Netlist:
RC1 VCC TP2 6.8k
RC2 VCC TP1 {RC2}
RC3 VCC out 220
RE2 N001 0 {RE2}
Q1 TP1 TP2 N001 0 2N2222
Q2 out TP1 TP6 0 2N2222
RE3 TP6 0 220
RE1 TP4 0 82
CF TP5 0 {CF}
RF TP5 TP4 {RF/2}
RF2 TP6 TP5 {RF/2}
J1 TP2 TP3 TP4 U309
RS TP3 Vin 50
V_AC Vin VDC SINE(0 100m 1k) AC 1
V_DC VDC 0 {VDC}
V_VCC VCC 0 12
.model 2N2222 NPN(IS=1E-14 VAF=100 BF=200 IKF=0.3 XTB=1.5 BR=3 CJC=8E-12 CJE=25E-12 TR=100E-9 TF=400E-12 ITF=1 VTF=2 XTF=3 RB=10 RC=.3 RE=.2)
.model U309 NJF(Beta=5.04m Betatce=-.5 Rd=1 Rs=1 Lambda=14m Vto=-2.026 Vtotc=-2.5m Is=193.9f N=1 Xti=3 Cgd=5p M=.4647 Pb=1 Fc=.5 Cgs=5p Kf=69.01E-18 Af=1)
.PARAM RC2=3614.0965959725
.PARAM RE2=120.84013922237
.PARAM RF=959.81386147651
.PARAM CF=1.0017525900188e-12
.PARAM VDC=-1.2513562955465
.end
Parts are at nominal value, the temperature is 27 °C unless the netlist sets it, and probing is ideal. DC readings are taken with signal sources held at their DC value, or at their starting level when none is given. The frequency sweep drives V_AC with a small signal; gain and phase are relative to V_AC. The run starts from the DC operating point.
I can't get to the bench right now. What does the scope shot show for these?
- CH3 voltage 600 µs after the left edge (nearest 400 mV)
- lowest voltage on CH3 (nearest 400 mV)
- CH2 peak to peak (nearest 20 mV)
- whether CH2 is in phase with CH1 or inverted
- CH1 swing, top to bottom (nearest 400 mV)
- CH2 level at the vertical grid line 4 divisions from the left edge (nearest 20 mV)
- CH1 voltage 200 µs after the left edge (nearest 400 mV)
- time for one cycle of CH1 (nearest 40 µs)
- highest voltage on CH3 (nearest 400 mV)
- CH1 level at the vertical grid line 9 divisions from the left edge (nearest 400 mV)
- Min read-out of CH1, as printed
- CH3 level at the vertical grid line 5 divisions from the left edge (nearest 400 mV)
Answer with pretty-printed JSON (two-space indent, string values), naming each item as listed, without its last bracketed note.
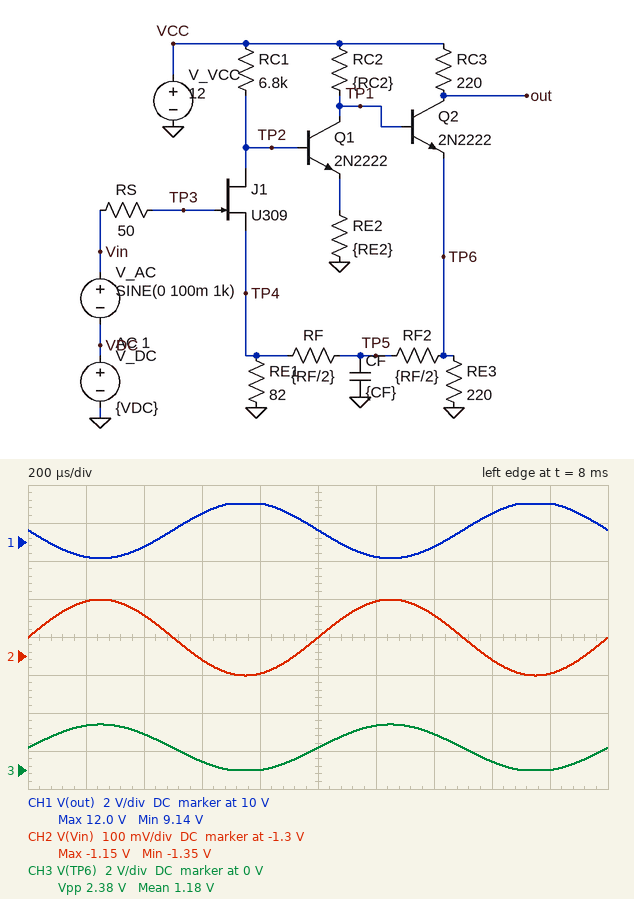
{
  "CH3 voltage 600 µs after the left edge": "400 mV",
  "lowest voltage on CH3": "0 V",
  "CH2 peak to peak": "200 mV",
  "whether CH2 is in phase with CH1 or inverted": "inverted",
  "CH1 swing, top to bottom": "2.8 V",
  "CH2 level at the vertical grid line 4 divisions from the left edge": "-1.34 V",
  "CH1 voltage 200 µs after the left edge": "9.2 V",
  "time for one cycle of CH1": "1.00 ms",
  "highest voltage on CH3": "2.4 V",
  "CH1 level at the vertical grid line 9 divisions from the left edge": "12.0 V",
  "Min read-out of CH1, as printed": "9.14 V",
  "CH3 level at the vertical grid line 5 divisions from the left edge": "1.2 V"
}
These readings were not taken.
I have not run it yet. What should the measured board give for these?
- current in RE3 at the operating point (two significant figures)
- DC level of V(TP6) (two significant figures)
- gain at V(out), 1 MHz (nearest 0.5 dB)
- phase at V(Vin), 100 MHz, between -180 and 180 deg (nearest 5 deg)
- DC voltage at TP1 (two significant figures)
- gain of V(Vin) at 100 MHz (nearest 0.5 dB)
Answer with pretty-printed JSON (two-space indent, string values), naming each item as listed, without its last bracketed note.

{
  "current in RE3 at the operating point": "5.3 mA",
  "DC level of V(TP6)": "1.2 V",
  "gain at V(out), 1 MHz": "23.5 dB",
  "phase at V(Vin), 100 MHz, between -180 and 180 deg": "0 deg",
  "DC voltage at TP1": "1.9 V",
  "gain of V(Vin) at 100 MHz": "0 dB"
}
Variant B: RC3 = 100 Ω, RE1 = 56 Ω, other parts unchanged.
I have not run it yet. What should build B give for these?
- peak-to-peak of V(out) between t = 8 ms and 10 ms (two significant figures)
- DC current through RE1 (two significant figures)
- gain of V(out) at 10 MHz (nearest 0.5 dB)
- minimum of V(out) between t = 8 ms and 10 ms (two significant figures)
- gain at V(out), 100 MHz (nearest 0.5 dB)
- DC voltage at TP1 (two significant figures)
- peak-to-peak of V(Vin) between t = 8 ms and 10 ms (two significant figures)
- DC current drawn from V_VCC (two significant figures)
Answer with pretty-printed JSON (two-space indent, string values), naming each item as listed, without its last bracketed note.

{
  "peak-to-peak of V(out) between t = 8 ms and 10 ms": "1.9 V",
  "DC current through RE1": "3.8 mA",
  "gain of V(out) at 10 MHz": "15.5 dB",
  "minimum of V(out) between t = 8 ms and 10 ms": "9.8 V",
  "gain at V(out), 100 MHz": "-8.5 dB",
  "DC voltage at TP1": "3.0 V",
  "peak-to-peak of V(Vin) between t = 8 ms and 10 ms": "200 mV",
  "DC current drawn from V_VCC": "17 mA"
}
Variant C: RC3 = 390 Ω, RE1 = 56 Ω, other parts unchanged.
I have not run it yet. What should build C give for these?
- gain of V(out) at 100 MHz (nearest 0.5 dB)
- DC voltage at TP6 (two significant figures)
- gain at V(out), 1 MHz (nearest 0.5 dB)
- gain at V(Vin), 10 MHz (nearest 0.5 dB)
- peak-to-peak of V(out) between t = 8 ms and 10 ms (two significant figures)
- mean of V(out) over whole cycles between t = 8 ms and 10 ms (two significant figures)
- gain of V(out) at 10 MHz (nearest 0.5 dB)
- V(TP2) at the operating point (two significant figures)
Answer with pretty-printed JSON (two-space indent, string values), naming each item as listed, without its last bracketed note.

{
  "gain of V(out) at 100 MHz": "-2.0 dB",
  "DC voltage at TP6": "2.3 V",
  "gain at V(out), 1 MHz": "31.5 dB",
  "gain at V(Vin), 10 MHz": "0 dB",
  "peak-to-peak of V(out) between t = 8 ms and 10 ms": "7.0 V",
  "mean of V(out) over whole cycles between t = 8 ms and 10 ms": "7.2 V",
  "gain of V(out) at 10 MHz": "27.0 dB",
  "V(TP2) at the operating point": "970 mV"
}
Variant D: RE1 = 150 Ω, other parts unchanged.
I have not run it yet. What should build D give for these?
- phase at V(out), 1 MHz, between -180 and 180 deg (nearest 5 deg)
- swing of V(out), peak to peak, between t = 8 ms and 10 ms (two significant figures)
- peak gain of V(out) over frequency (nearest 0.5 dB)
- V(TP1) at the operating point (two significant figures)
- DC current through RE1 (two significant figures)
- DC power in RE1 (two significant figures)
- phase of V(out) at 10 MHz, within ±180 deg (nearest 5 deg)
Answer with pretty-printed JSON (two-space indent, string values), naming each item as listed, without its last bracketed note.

{
  "phase at V(out), 1 MHz, between -180 and 180 deg": "155 deg",
  "swing of V(out), peak to peak, between t = 8 ms and 10 ms": "880 mV",
  "peak gain of V(out) over frequency": "18.5 dB",
  "V(TP1) at the operating point": "650 mV",
  "DC current through RE1": "1.4 mA",
  "DC power in RE1": "310 µW",
  "phase of V(out) at 10 MHz, within ±180 deg": "50 deg"
}
